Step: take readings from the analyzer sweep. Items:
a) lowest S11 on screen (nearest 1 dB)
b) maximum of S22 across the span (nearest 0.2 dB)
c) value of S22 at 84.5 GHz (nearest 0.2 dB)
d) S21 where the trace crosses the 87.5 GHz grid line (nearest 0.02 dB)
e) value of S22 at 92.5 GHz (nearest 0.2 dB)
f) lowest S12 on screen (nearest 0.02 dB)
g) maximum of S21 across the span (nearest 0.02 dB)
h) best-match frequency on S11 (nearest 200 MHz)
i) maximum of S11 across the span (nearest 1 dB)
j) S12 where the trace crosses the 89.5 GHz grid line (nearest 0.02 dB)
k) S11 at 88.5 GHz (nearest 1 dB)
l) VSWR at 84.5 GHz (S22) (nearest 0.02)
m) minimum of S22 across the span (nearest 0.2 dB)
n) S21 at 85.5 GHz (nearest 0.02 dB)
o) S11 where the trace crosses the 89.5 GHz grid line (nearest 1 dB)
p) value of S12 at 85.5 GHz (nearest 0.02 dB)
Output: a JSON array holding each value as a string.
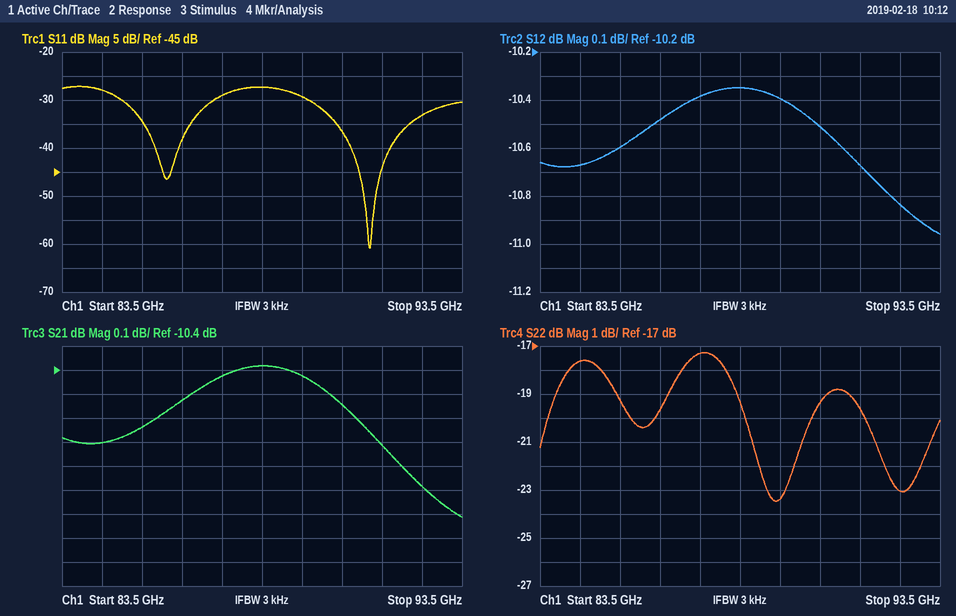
["-61 dB", "-17.2 dB", "-17.6 dB", "-10.42 dB", "-23.0 dB", "-10.96 dB", "-10.38 dB", "91.2 GHz", "-27 dB", "-10.40 dB", "-27 dB", "1.30", "-23.4 dB", "-10.64 dB", "-29 dB", "-10.60 dB"]
